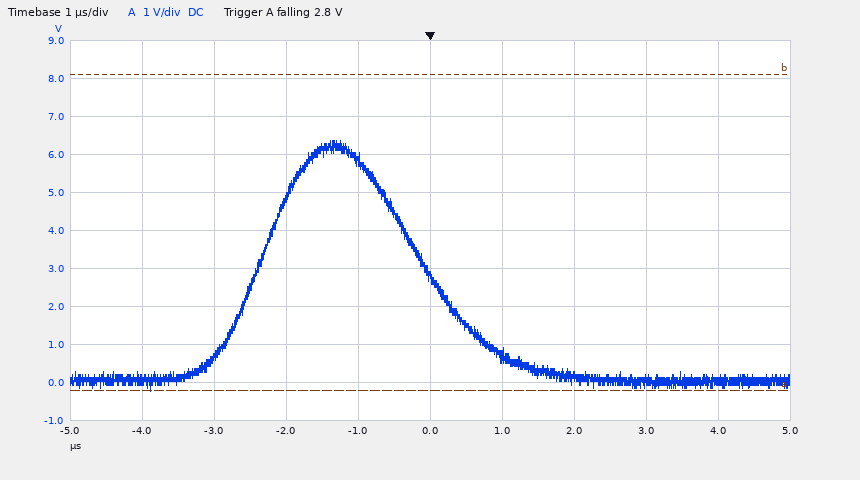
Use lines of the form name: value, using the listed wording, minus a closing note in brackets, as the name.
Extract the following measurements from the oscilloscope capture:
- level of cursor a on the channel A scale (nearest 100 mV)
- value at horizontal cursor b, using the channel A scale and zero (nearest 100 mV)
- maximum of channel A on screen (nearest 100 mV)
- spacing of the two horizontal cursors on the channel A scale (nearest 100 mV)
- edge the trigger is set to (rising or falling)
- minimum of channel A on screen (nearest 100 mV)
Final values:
level of cursor a on the channel A scale: -200 mV
value at horizontal cursor b, using the channel A scale and zero: 8.1 V
maximum of channel A on screen: 6.4 V
spacing of the two horizontal cursors on the channel A scale: 8.3 V
edge the trigger is set to: falling
minimum of channel A on screen: -200 mV
